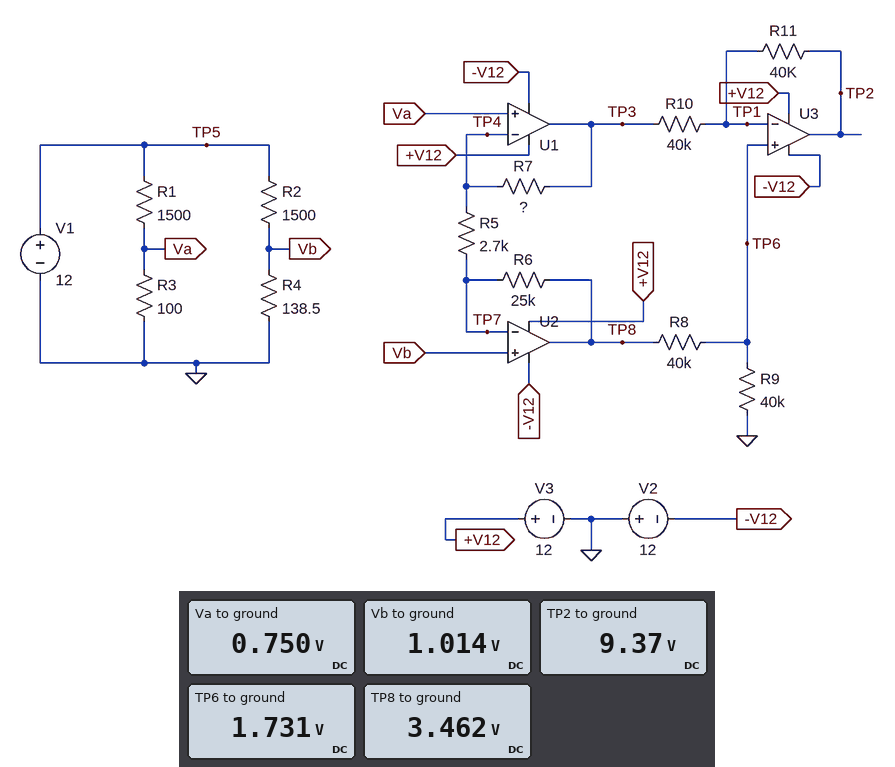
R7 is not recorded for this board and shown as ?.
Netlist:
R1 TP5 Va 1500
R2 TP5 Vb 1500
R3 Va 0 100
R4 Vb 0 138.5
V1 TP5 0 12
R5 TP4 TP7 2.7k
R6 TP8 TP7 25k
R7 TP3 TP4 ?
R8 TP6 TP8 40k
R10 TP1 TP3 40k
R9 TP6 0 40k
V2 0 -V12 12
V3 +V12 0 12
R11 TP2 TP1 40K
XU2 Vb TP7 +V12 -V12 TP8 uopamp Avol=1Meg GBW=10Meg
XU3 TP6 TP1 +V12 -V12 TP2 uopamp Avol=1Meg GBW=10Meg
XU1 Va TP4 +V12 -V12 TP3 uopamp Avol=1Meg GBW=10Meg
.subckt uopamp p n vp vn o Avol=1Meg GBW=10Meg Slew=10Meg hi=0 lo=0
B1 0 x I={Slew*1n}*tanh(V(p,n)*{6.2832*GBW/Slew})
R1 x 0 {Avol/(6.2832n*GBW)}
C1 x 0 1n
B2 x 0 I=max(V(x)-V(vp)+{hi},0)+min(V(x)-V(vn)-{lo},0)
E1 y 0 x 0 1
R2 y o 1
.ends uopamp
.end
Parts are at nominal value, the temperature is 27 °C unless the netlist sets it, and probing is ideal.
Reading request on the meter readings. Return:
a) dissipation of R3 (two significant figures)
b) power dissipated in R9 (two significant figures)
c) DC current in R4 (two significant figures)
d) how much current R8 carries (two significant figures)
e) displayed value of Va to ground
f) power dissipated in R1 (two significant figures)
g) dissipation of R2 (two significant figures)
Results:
5.6 mW
75 µW
7.3 mA
43 µA
0.750 V
84 mW
80 mW
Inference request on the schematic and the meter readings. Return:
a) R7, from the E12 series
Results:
68 kΩ
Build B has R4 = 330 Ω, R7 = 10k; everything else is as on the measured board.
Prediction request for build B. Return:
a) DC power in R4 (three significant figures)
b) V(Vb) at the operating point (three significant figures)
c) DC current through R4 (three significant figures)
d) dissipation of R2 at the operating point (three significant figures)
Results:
14.2 mW
2.16 V
6.56 mA
64.5 mW
